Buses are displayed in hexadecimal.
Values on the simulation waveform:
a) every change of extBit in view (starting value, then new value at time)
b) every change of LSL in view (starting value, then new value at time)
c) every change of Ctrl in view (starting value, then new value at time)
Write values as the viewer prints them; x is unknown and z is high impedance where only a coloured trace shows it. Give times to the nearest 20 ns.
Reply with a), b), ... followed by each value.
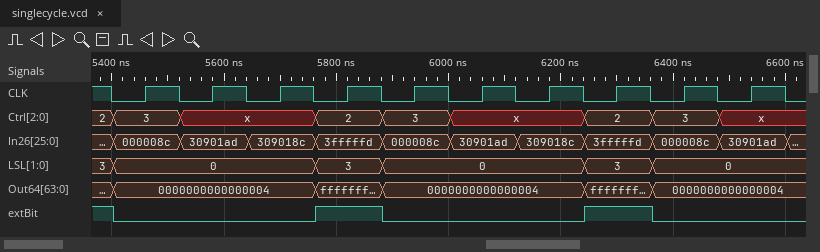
a) 1, 0 at 5400 ns, 1 at 5760 ns, 0 at 5880 ns, 1 at 6240 ns, 0 at 6360 ns
b) 3, 0 at 5400 ns, 3 at 5760 ns, 0 at 5880 ns, 3 at 6240 ns, 0 at 6360 ns
c) 2, 3 at 5400 ns, x at 5520 ns, 2 at 5760 ns, 3 at 5880 ns, x at 6000 ns, 2 at 6240 ns, 3 at 6360 ns, x at 6480 ns
